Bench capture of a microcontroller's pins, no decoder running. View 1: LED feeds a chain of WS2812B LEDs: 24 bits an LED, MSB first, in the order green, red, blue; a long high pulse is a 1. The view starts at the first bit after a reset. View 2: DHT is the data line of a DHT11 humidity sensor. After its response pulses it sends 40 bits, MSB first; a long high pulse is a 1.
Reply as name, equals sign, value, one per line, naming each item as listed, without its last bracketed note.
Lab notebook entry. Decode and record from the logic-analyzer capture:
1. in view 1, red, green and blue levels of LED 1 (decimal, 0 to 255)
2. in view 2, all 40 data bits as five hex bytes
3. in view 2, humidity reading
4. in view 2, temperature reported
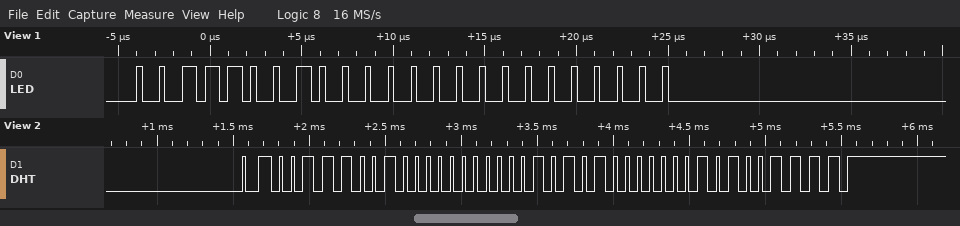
in view 1, red, green and blue levels of LED 1 = 0, 57, 0
in view 2, all 40 data bits as five hex bytes = 39 00 15 01 4F
in view 2, humidity reading = 57 %
in view 2, temperature reported = 21.1 °C
